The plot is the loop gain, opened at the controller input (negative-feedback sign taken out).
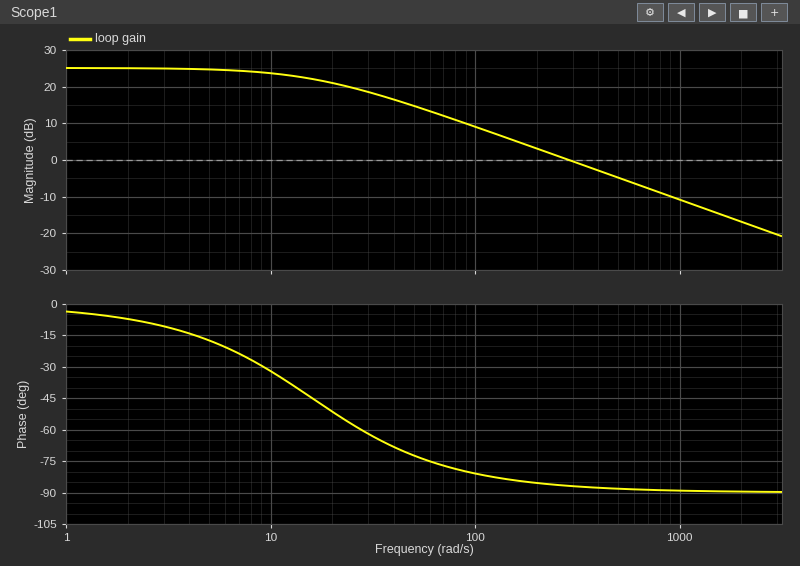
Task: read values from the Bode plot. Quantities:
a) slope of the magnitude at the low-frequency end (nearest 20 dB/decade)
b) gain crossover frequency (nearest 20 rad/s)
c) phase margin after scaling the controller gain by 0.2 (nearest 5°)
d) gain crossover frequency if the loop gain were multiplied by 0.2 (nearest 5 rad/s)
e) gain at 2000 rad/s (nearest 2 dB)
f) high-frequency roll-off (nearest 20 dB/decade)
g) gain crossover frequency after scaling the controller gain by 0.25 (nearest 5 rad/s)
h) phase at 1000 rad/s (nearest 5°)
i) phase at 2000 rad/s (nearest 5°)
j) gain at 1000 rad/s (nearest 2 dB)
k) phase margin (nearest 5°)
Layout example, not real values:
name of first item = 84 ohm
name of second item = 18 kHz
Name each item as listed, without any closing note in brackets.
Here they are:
slope of the magnitude at the low-frequency end = 0 dB/decade
gain crossover frequency = 280 rad/s
phase margin after scaling the controller gain by 0.2 = 105°
gain crossover frequency if the loop gain were multiplied by 0.2 = 55 rad/s
gain at 2000 rad/s = -16 dB
high-frequency roll-off = -20 dB/decade
gain crossover frequency after scaling the controller gain by 0.25 = 70 rad/s
phase at 1000 rad/s = -90°
phase at 2000 rad/s = -90°
gain at 1000 rad/s = -10 dB
phase margin = 95°
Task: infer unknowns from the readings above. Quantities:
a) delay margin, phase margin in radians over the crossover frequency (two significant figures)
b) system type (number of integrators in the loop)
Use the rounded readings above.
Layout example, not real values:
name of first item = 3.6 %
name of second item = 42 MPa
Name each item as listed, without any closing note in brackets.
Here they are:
delay margin, phase margin in radians over the crossover frequency = 0.0059 s
system type = 0
